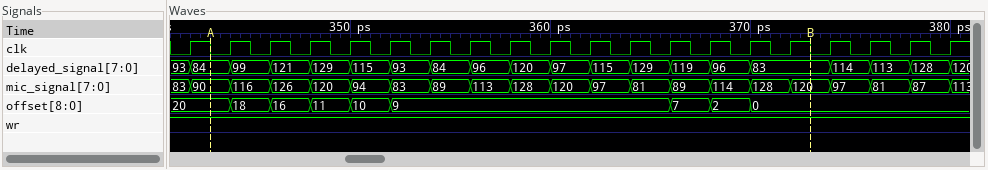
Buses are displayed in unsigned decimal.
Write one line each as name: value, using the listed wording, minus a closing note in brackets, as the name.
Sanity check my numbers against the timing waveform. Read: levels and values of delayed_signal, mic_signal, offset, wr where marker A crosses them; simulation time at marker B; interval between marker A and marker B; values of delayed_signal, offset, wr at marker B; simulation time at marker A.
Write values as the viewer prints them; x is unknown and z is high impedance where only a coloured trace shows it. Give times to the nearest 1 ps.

levels and values of delayed_signal, mic_signal, offset, wr where marker A crosses them: delayed_signal=84, mic_signal=90, offset=20, wr=1
simulation time at marker B: 373 ps
interval between marker A and marker B: 30 ps
values of delayed_signal, offset, wr at marker B: delayed_signal=83, offset=0, wr=1
simulation time at marker A: 343 ps
